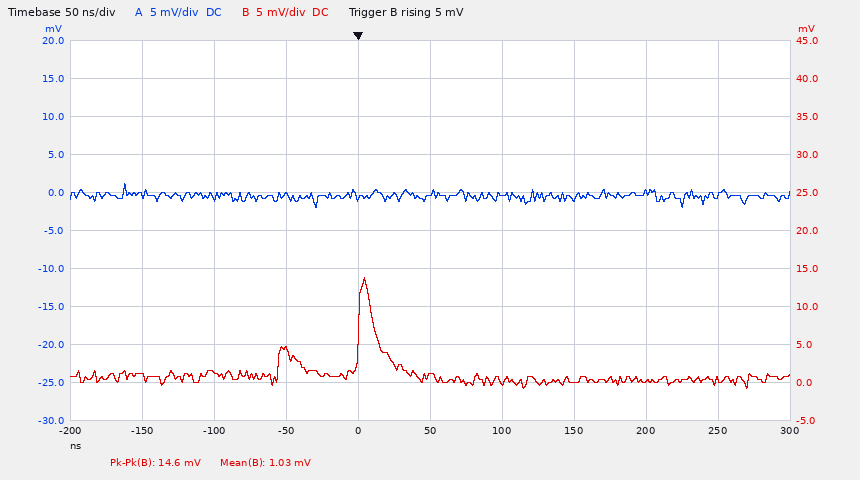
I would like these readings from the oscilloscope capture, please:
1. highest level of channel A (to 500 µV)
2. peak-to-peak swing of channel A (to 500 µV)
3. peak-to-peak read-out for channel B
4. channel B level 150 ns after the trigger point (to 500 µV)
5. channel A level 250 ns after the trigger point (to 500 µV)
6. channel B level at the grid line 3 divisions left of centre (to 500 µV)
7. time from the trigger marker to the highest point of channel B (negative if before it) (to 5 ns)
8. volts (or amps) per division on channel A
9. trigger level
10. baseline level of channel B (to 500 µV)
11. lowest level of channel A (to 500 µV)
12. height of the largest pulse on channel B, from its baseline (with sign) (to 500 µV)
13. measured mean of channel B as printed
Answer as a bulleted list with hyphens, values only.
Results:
- 1.0 mV
- 3.0 mV
- 14.6 mV
- 0.0 mV
- -500 µV
- 1.5 mV
- +5 ns
- 5 mV
- 5 mV
- 500 µV
- -2.0 mV
- +13.0 mV
- 1.03 mV
